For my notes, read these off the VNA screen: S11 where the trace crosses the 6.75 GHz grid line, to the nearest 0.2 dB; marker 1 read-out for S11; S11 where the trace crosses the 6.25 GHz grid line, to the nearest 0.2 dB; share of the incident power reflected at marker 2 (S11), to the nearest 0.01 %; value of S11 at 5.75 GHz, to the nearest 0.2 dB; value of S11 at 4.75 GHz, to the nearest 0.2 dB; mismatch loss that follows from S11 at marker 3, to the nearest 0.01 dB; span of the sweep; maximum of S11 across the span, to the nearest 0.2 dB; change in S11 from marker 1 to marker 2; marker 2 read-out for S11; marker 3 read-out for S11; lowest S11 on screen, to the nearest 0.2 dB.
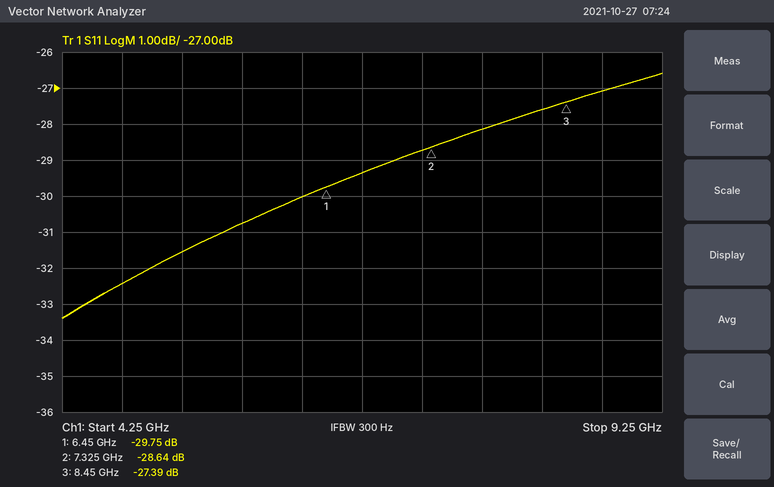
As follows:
-29.4 dB
-29.75 dB
-30.0 dB
0.14 %
-30.8 dB
-32.4 dB
0.01 dB
5 GHz
-26.6 dB
1.11 dB
-28.64 dB
-27.39 dB
-33.4 dB
